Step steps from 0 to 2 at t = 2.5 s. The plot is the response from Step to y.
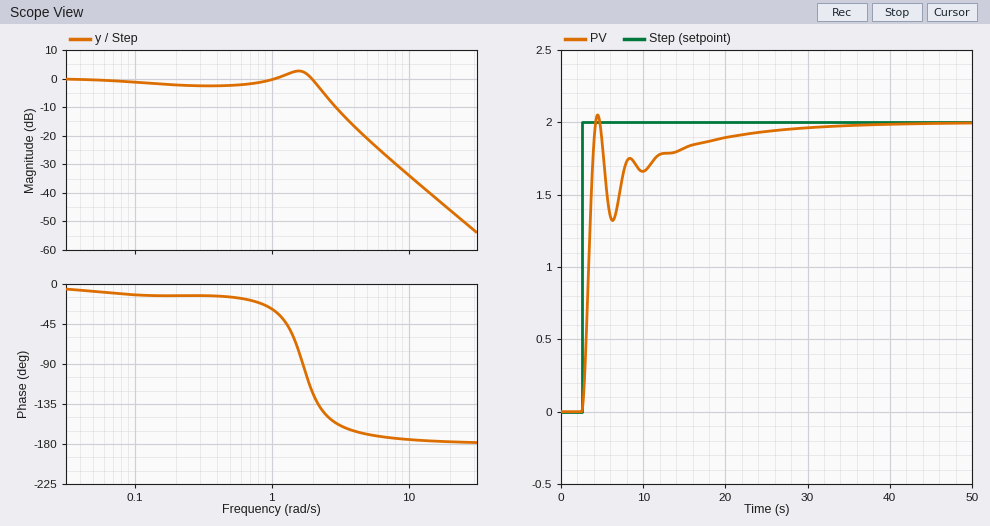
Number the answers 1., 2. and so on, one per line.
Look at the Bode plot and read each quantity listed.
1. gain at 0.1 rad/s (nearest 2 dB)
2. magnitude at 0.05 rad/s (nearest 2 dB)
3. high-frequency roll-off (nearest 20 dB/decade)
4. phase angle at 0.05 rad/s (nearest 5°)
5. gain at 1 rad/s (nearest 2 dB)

1. -2 dB
2. 0 dB
3. -40 dB/decade
4. -10°
5. 0 dB
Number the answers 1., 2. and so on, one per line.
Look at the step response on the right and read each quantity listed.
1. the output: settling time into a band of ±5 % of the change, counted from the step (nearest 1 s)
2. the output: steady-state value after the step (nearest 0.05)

1. 18 s
2. 2.00
